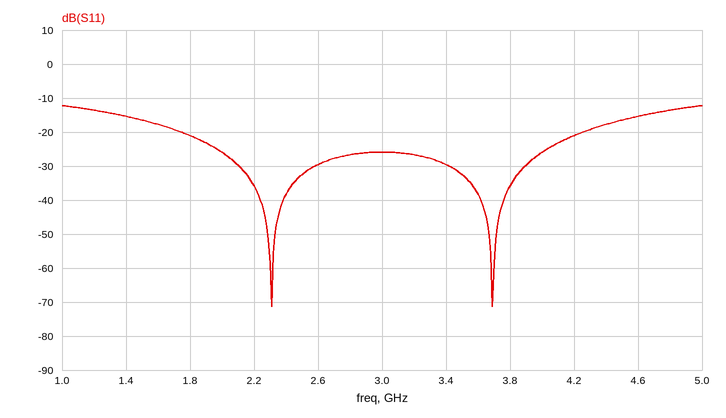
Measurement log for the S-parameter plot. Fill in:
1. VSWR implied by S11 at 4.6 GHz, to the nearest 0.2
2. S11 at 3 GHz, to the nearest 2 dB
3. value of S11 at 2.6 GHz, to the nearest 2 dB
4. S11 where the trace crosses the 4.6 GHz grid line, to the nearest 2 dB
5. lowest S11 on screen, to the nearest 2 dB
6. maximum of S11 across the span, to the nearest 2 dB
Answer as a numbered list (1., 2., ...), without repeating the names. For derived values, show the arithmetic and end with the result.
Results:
1. |Γ| = 10^(-16/20) = 0.1585; VSWR = (1 + 0.1585)/(1 − 0.1585) ≈ 1.4
2. -26 dB
3. -30 dB
4. -16 dB
5. -72 dB
6. -12 dB
